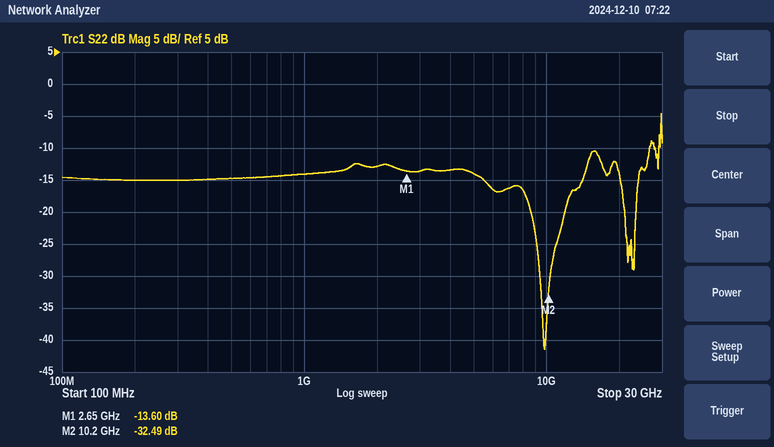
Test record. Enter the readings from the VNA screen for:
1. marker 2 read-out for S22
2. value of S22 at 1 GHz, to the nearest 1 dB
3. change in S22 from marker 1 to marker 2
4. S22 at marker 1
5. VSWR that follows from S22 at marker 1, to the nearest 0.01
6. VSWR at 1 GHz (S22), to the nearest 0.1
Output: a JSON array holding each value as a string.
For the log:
["-32.49 dB", "-14 dB", "-18.89 dB", "-13.60 dB", "1.53", "1.5"]
